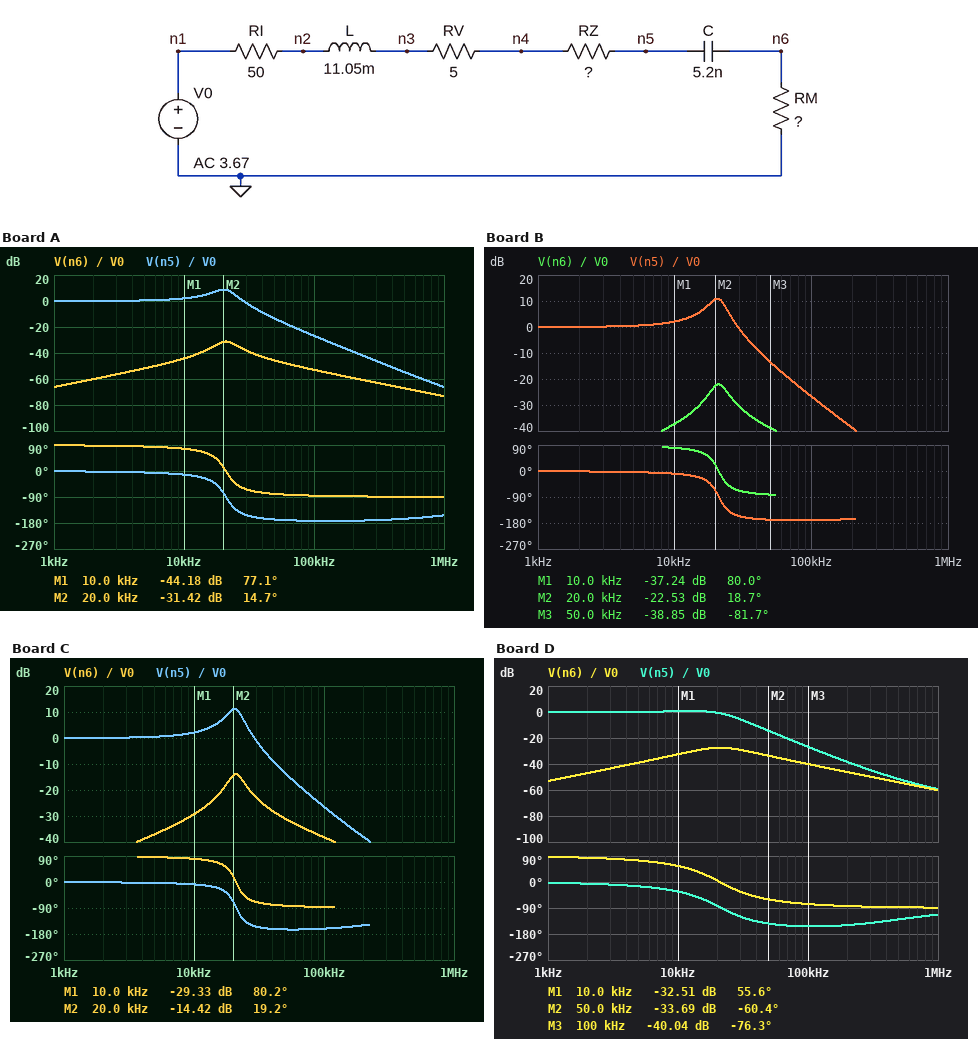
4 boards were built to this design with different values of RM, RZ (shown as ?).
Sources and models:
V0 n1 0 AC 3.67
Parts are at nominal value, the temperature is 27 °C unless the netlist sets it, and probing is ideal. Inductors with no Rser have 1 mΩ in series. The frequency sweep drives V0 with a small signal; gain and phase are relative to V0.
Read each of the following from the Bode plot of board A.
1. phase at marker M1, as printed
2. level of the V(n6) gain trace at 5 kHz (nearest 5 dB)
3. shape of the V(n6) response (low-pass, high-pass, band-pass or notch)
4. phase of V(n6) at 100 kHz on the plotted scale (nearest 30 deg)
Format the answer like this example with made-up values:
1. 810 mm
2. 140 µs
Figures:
1. 77.1 deg
2. -50 dB
3. band-pass
4. -90 deg
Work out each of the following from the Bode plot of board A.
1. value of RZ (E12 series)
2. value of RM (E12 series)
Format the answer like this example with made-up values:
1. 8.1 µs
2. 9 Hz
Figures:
1. 470 Ω
2. 15 Ω
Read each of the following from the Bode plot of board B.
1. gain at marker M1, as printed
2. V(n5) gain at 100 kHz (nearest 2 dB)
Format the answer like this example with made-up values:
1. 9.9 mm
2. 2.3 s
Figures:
1. -37.24 dB
2. -26 dB
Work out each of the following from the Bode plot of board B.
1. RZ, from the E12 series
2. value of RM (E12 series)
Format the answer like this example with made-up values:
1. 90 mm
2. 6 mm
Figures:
1. 330 Ω
2. 33 Ω
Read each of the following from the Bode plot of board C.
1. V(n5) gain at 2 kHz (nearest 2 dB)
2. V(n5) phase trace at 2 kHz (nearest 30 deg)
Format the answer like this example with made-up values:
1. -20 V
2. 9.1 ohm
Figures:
1. 0 dB
2. 0 deg
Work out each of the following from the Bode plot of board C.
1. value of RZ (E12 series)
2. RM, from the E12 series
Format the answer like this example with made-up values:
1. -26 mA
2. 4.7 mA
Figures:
1. 270 Ω
2. 82 Ω
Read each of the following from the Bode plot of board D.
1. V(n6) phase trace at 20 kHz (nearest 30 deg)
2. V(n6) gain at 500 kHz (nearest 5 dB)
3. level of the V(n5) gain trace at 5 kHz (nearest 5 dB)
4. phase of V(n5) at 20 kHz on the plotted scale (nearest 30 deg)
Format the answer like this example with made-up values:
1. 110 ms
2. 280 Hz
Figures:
1. 0 deg
2. -55 dB
3. 0 dB
4. -90 deg
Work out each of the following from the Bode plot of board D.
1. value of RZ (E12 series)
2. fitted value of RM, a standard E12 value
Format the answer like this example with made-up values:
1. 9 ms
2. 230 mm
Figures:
1. 1.5 kΩ
2. 68 Ω
